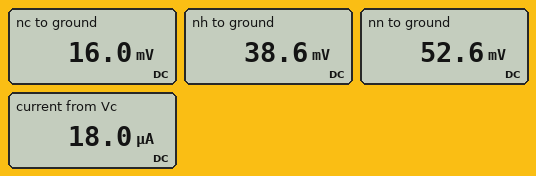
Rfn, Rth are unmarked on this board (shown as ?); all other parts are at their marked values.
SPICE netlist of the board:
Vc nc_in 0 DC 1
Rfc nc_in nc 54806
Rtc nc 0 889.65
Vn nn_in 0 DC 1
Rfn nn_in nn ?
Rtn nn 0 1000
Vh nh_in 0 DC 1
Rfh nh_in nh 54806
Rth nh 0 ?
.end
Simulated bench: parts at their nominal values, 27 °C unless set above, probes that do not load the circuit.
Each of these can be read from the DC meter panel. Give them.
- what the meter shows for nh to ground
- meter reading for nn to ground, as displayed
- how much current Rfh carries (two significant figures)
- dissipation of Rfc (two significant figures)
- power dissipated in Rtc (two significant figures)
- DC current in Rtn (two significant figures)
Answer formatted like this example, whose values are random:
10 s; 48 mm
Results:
38.6 mV; 52.6 mV; 18 µA; 18 µW; 290 nW; 53 µA
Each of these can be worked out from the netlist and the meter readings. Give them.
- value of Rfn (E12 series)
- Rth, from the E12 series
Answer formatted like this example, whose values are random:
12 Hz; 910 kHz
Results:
18 kΩ; 2.2 kΩ
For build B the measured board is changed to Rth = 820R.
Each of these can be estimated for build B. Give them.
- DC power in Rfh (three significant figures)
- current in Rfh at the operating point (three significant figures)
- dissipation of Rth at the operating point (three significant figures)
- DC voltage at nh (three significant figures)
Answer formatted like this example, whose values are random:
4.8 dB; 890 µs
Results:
17.7 µW; 18.0 µA; 265 nW; 14.7 mV
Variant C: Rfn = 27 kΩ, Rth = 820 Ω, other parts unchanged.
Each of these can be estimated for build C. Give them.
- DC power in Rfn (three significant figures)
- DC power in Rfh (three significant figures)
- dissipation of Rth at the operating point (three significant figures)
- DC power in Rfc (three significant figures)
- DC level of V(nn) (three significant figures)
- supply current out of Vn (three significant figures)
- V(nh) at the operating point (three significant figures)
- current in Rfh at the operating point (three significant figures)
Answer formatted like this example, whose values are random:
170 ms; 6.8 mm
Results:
34.4 µW; 17.7 µW; 265 nW; 17.7 µW; 35.7 mV; 35.7 µA; 14.7 mV; 18.0 µA
